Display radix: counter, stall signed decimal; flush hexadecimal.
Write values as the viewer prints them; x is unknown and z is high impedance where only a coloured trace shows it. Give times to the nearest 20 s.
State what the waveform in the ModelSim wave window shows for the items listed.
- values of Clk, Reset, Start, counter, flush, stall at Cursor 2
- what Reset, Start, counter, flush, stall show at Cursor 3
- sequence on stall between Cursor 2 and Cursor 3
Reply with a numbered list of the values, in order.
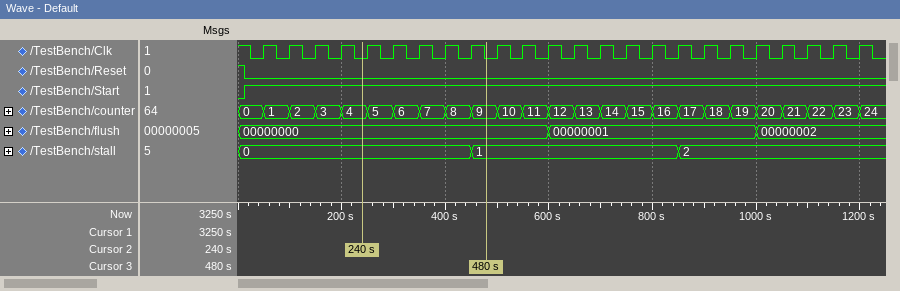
1. Clk=0, Reset=0, Start=1, counter=4, flush=00000000, stall=0
2. Reset=0, Start=1, counter=9, flush=00000000, stall=1
3. 0, 1
